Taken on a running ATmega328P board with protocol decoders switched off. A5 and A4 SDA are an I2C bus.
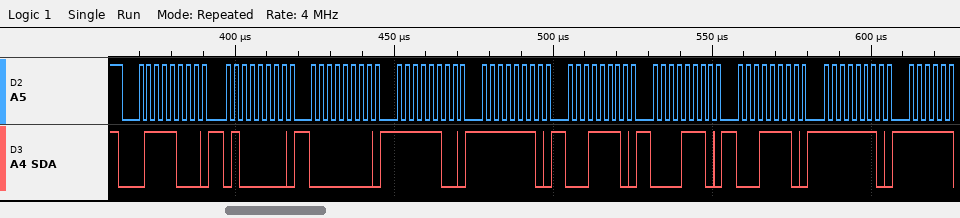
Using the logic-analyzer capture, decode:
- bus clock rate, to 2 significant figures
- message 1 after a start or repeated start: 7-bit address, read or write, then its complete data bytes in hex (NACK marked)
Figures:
400 kHz
0x3C write: 40 00 FC FE 1E 0E 1E FE
